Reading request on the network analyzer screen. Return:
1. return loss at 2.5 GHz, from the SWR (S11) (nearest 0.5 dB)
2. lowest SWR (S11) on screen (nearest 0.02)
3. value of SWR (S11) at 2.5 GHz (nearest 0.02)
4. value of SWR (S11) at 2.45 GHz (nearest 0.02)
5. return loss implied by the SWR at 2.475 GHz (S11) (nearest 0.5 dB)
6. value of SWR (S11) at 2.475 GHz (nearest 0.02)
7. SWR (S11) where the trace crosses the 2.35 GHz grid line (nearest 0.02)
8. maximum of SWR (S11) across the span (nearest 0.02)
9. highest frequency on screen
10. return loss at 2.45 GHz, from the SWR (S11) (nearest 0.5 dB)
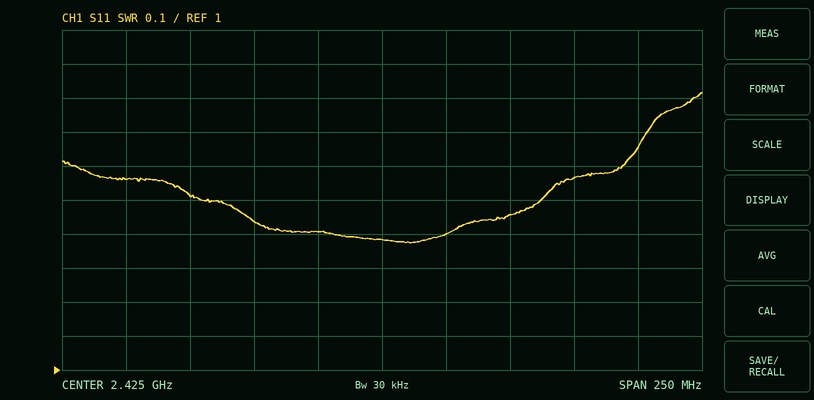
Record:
13.0 dB
1.38
1.56
1.40
14.5 dB
1.46
1.52
1.82
2.55 GHz
15.5 dB
